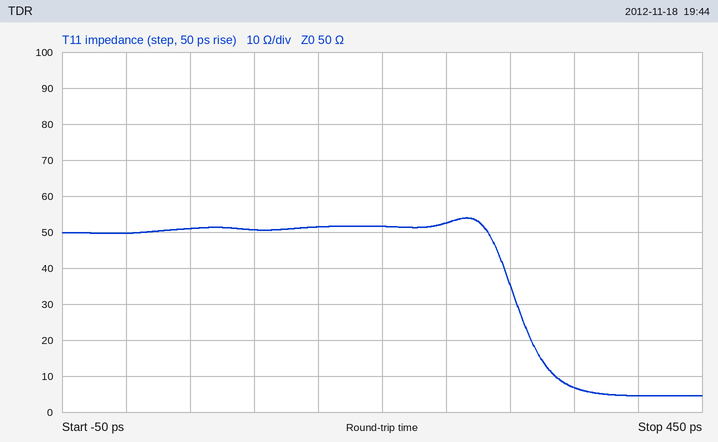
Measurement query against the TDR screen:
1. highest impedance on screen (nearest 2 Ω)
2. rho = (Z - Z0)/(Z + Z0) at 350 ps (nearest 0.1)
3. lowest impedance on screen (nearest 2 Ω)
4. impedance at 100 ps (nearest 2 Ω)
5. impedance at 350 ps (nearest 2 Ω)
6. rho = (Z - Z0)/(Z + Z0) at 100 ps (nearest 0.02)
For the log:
54 Ω
-0.8
4 Ω
50 Ω
6 Ω
0.00
